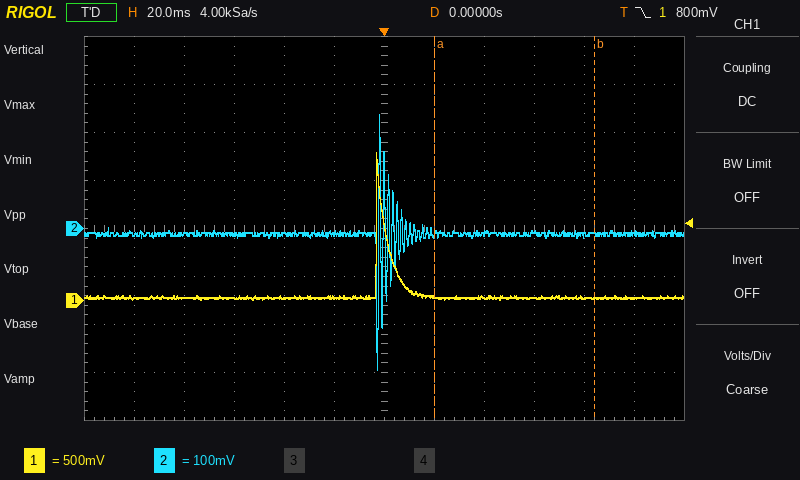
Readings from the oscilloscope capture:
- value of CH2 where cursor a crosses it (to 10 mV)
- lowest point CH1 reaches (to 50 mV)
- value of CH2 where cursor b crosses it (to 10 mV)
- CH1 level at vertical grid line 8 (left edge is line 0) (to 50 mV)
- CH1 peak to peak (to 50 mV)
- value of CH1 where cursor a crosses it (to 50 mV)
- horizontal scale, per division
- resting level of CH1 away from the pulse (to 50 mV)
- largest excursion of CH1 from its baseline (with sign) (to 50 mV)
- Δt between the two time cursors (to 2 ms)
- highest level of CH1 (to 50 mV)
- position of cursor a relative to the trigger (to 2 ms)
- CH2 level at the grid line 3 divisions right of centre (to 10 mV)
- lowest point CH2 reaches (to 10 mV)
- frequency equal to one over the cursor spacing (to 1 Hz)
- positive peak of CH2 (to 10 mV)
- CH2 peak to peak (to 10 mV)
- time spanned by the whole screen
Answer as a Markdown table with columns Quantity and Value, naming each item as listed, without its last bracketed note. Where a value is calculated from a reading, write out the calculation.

| Quantity | Value |
|---|---|
| value of CH2 where cursor a crosses it | -10 mV |
| lowest point CH1 reaches | 0 mV |
| value of CH2 where cursor b crosses it | -10 mV |
| CH1 level at vertical grid line 8 (left edge is line 0) | 50 mV |
| CH1 peak to peak | 1.55 V − (0 mV) = 1.55 V |
| value of CH1 where cursor a crosses it | 50 mV |
| horizontal scale, per division | 20 ms |
| resting level of CH1 away from the pulse | 50 mV |
| largest excursion of CH1 from its baseline (with sign) | 1.55 V − (50 mV) = +1.50 V |
| Δt between the two time cursors | 64 ms |
| highest level of CH1 | 1.55 V |
| position of cursor a relative to the trigger | +20 ms |
| CH2 level at the grid line 3 divisions right of centre | -10 mV |
| lowest point CH2 reaches | -290 mV |
| frequency equal to one over the cursor spacing | 1 / 64 ms ≈ 16 Hz |
| positive peak of CH2 | 240 mV |
| CH2 peak to peak | 240 mV − (-290 mV) = 530 mV |
| time spanned by the whole screen | 240 ms |
